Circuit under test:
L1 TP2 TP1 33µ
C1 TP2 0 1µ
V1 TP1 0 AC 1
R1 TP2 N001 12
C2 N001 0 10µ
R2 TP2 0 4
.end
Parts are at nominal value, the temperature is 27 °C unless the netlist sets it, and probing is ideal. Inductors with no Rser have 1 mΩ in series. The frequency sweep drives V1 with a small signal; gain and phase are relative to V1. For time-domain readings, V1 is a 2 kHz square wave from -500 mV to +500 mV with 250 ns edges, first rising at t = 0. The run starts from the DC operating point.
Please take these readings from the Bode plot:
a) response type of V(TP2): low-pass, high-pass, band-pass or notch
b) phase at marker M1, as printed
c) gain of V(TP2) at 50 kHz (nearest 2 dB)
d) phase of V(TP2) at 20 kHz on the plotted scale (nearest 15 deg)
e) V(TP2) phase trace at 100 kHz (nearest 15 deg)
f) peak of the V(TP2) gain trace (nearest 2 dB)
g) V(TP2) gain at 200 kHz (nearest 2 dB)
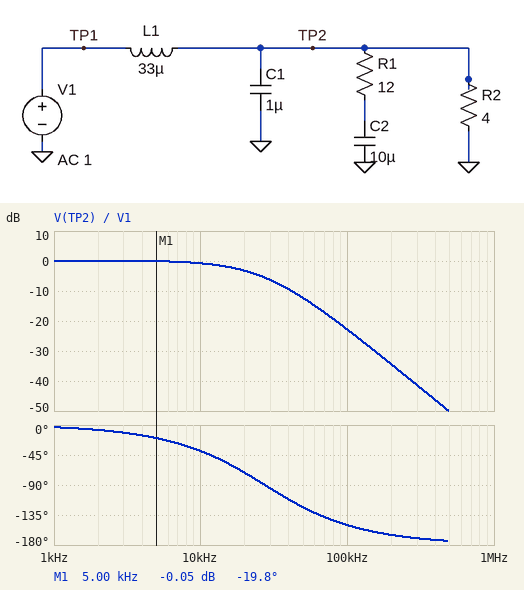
low-pass
-19.8 deg
-12 dB
-75 deg
-150 deg
0 dB
-34 dB
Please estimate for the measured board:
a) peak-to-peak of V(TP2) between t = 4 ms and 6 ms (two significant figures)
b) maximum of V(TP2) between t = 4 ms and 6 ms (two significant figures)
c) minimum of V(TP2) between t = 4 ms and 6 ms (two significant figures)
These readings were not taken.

1.0 V
520 mV
-520 mV
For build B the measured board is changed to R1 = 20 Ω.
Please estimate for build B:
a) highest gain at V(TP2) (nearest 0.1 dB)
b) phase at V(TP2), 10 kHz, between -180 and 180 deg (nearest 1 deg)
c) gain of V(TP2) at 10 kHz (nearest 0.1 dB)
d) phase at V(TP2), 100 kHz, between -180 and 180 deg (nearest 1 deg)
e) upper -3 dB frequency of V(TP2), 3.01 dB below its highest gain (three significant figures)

0 dB
-36 deg
-0.5 dB
-153 deg
21.8 kHz
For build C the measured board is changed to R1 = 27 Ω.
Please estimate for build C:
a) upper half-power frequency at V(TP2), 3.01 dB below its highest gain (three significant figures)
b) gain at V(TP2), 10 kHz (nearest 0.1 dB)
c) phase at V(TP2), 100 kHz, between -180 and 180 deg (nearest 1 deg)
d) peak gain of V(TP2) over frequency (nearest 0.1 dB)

23.2 kHz
-0.4 dB
-154 deg
0 dB
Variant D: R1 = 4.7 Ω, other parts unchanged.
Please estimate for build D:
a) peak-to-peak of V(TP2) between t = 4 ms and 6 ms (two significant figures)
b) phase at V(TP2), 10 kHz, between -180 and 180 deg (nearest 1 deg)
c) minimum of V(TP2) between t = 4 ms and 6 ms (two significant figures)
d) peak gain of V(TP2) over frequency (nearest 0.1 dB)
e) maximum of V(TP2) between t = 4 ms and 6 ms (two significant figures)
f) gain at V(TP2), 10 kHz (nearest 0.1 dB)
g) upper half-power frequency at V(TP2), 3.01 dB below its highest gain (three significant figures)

1.1 V
-51 deg
-570 mV
0.5 dB
570 mV
-1.4 dB
12.5 kHz
